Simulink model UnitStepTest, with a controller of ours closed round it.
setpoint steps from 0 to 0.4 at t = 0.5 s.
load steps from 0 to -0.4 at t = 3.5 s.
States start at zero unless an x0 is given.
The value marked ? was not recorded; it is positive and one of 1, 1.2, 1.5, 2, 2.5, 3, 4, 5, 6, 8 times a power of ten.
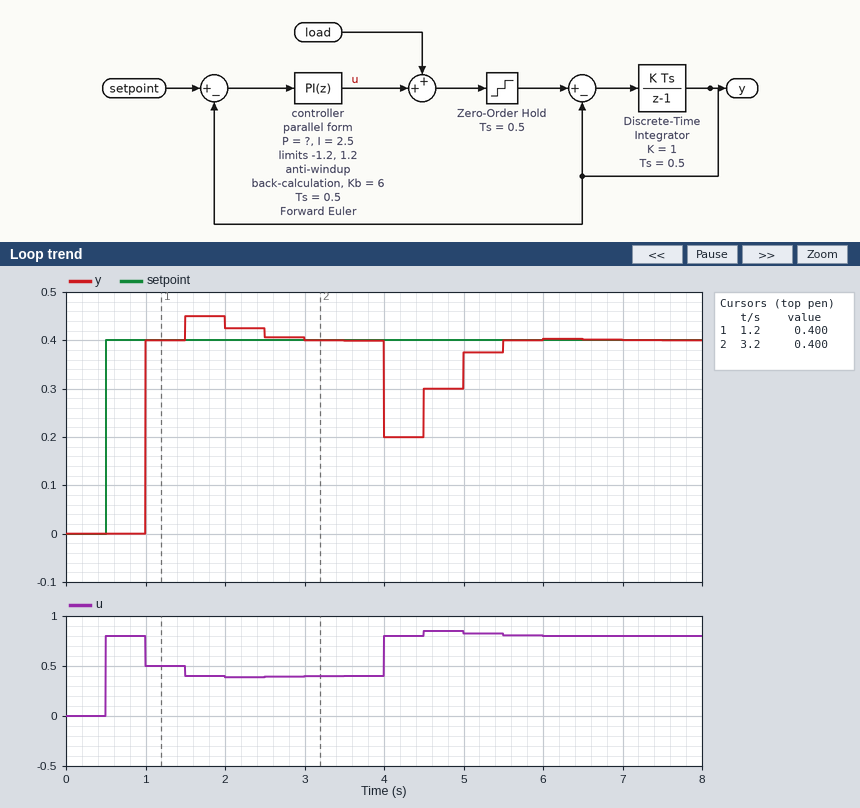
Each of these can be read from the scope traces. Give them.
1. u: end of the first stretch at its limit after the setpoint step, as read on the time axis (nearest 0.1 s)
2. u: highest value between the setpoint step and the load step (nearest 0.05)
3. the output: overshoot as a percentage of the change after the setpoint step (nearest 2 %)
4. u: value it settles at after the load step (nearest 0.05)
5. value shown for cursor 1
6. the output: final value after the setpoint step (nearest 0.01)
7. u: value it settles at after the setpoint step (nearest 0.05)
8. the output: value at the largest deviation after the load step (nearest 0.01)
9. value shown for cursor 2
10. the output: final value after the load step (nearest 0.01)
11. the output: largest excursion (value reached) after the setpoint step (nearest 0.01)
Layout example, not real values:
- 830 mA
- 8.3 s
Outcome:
- 1.0 s
- 0.80
- 12 %
- 0.80
- 0.400
- 0.40
- 0.40
- 0.20
- 0.400
- 0.40
- 0.45
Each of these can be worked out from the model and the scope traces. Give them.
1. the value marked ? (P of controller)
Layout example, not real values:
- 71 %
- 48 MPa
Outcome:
- 2
